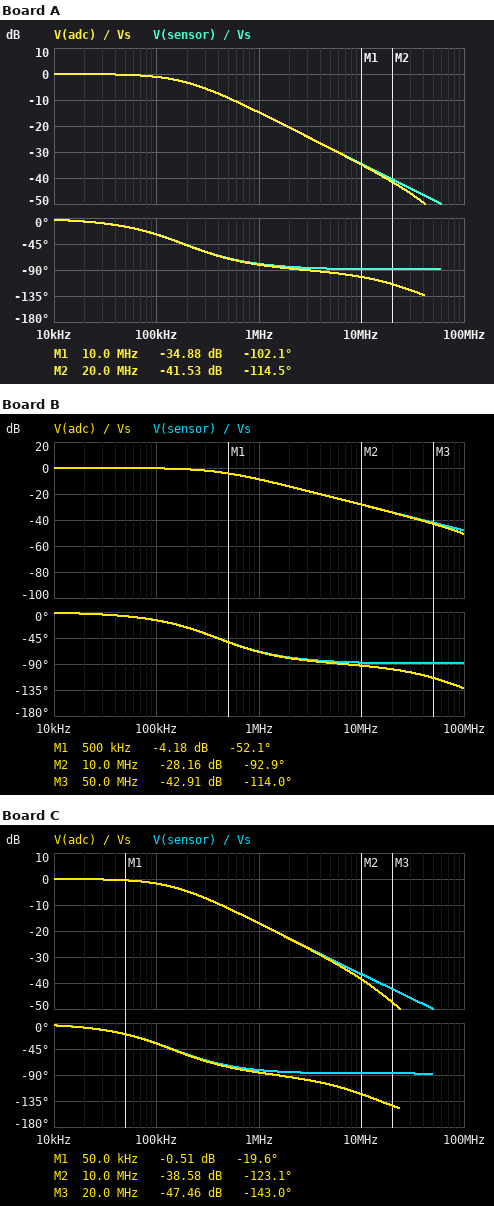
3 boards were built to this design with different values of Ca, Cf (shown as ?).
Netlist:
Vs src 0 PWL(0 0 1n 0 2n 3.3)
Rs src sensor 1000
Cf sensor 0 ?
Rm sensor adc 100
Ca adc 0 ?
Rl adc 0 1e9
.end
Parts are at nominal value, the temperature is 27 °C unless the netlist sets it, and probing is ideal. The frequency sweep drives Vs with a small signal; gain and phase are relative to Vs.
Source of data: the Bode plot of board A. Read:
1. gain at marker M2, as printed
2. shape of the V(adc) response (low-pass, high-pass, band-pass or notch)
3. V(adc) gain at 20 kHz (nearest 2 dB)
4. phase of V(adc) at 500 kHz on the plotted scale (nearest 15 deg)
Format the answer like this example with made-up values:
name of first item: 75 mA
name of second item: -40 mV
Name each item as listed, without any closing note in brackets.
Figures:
gain at marker M2, as printed: -41.53 dB
shape of the V(adc) response: low-pass
V(adc) gain at 20 kHz: 0 dB
phase of V(adc) at 500 kHz on the plotted scale: -75 deg
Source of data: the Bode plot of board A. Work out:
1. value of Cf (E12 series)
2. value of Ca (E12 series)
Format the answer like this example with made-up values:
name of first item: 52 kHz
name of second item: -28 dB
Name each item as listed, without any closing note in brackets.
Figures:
value of Cf: 820 pF
value of Ca: 39 pF
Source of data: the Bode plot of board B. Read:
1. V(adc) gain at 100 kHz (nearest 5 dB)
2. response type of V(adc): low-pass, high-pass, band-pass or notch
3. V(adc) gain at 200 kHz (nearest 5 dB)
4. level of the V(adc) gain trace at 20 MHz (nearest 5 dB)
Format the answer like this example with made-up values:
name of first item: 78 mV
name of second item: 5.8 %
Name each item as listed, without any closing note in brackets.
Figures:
V(adc) gain at 100 kHz: 0 dB
response type of V(adc): low-pass, high-pass, band-pass or notch: low-pass
V(adc) gain at 200 kHz: 0 dB
level of the V(adc) gain trace at 20 MHz: -35 dB
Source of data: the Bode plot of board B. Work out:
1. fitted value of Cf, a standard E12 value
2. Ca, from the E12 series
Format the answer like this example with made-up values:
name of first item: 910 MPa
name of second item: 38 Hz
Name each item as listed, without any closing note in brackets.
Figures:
fitted value of Cf, a standard E12 value: 390 pF
Ca, from the E12 series: 15 pF
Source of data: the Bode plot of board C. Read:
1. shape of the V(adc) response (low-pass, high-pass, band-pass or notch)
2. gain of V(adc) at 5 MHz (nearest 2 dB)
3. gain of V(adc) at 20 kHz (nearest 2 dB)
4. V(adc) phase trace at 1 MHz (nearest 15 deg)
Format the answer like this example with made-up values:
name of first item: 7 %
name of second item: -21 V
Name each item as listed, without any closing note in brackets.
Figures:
shape of the V(adc) response: low-pass
gain of V(adc) at 5 MHz: -32 dB
gain of V(adc) at 20 kHz: 0 dB
V(adc) phase trace at 1 MHz: -90 deg
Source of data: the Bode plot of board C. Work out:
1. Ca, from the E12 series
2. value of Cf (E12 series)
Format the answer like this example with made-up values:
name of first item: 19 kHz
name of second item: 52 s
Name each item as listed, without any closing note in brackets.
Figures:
Ca, from the E12 series: 120 pF
value of Cf: 1 nF
